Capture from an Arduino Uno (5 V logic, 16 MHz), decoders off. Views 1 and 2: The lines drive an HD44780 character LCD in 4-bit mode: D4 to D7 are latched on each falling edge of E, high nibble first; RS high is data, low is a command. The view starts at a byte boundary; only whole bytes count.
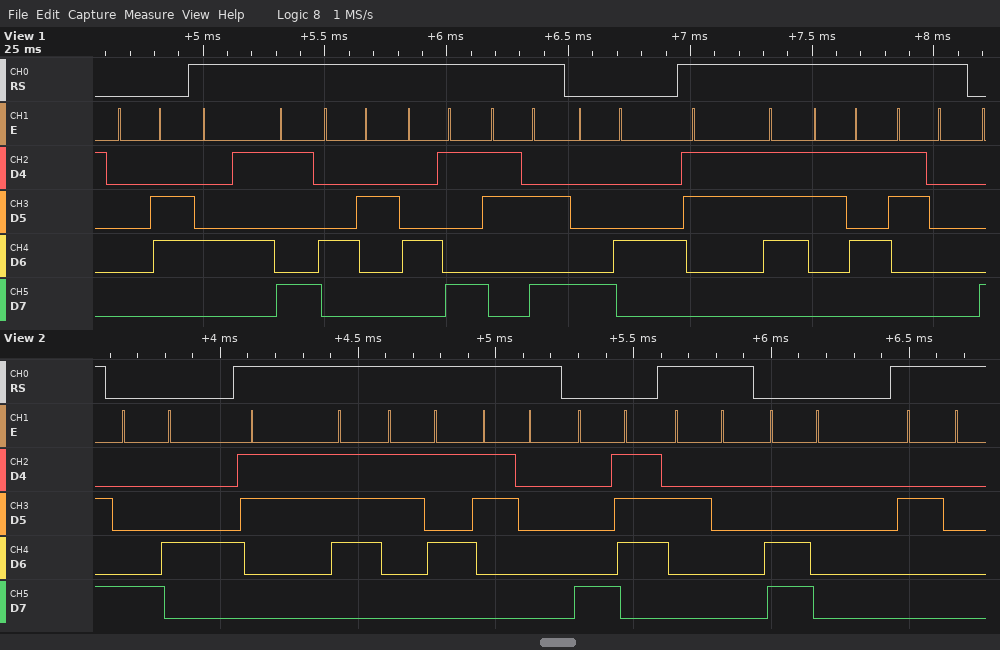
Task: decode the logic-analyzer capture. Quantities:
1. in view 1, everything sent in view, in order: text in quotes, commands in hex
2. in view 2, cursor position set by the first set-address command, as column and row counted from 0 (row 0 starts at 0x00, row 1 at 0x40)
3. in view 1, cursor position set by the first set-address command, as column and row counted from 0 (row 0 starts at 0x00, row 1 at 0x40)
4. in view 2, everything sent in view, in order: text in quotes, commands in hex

0x06 "IBI:" 0x84 "750"
column 4, row 0
column 4, row 0
0x84 "750" 0x87 " " 0xC0 " "
